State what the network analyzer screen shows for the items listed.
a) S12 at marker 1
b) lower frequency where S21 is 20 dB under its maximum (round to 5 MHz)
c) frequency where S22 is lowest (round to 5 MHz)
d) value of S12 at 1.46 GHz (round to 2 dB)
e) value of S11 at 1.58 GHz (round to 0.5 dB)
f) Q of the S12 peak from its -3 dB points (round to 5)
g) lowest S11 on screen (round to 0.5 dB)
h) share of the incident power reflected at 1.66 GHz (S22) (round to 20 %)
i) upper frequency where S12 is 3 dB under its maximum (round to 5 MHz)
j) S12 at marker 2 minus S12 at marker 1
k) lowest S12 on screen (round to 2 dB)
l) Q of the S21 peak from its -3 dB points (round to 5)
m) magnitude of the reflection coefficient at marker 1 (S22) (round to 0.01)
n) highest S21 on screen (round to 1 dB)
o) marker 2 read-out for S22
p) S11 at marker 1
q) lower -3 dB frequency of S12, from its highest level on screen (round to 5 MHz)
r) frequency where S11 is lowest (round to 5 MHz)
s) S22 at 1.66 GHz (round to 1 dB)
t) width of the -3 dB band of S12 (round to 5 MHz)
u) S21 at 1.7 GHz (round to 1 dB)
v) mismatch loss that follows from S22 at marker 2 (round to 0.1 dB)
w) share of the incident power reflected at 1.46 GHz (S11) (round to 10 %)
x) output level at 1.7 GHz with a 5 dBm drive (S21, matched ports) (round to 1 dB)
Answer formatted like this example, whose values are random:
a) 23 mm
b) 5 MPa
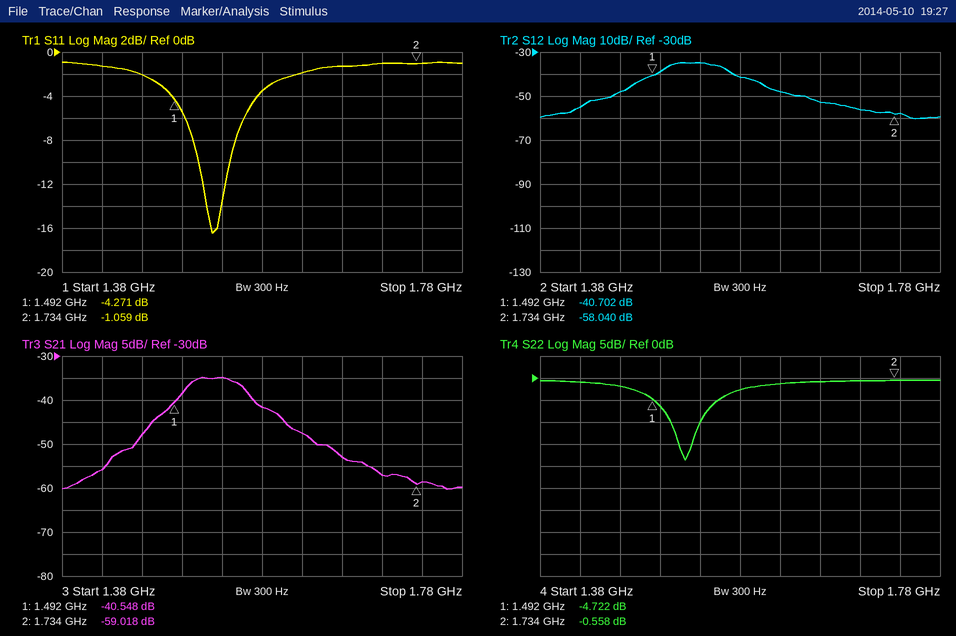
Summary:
a) -40.702 dB
b) 1.425 GHz
c) 1.525 GHz
d) -48 dB
e) -3.5 dB
f) 25
g) -16.5 dB
h) 80 %
i) 1.565 GHz
j) -17.338 dB
k) -60 dB
l) 25
m) 0.58
n) -35 dB
o) -0.558 dB
p) -4.271 dB
q) 1.505 GHz
r) 1.530 GHz
s) -1 dB
t) 60 MHz
u) -57 dB
v) 9.2 dB
w) 60 %
x) -52 dBm
